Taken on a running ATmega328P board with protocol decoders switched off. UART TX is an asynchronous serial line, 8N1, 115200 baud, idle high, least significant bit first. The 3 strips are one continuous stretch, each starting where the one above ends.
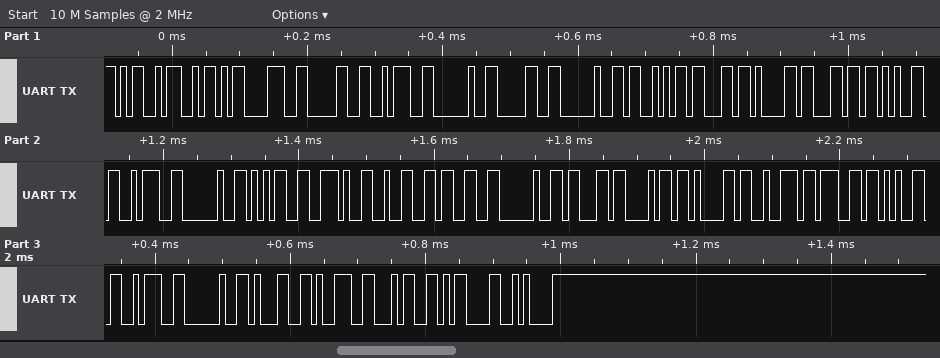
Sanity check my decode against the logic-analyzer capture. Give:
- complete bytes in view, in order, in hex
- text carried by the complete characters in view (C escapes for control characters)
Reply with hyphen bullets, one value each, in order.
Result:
- 4D 5A 38 30 3A 20 30 20 53 63 61 6C 65 3A 20 35 2E 32 33 20 63 68 61 72 67 65 3A 20 31 39 34 0D 0A
- "MZ80: 0 Scale: 5.23 charge: 194\r\n"
